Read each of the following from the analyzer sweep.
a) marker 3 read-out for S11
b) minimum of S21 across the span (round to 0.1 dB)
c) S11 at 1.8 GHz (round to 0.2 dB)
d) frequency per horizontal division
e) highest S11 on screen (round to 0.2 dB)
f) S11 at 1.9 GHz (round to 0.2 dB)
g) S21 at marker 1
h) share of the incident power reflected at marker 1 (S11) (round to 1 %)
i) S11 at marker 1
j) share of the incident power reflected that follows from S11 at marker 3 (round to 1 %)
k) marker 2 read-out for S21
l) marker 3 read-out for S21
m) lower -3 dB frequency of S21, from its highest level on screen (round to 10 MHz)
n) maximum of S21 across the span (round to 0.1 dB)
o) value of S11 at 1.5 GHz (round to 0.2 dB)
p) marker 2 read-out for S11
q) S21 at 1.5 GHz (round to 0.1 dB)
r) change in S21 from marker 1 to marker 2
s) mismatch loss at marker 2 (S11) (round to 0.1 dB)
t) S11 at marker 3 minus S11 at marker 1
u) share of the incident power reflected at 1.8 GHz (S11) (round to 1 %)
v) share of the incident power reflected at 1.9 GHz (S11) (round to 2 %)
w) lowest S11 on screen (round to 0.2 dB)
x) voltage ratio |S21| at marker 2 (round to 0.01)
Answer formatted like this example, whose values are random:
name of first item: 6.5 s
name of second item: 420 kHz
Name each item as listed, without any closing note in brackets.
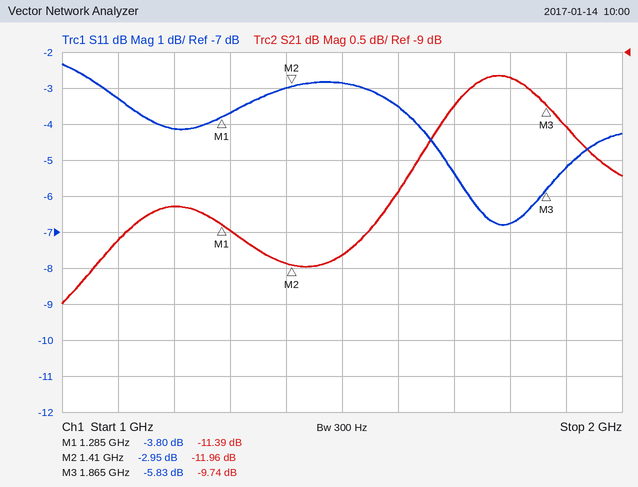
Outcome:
marker 3 read-out for S11: -5.83 dB
minimum of S21 across the span: -12.5 dB
S11 at 1.8 GHz: -6.8 dB
frequency per horizontal division: 100 MHz
highest S11 on screen: -2.4 dB
S11 at 1.9 GHz: -5.2 dB
S21 at marker 1: -11.39 dB
share of the incident power reflected at marker 1 (S11): 42 %
S11 at marker 1: -3.80 dB
share of the incident power reflected that follows from S11 at marker 3: 26 %
marker 2 read-out for S21: -11.96 dB
marker 3 read-out for S21: -9.74 dB
lower -3 dB frequency of S21, from its highest level on screen: 1.02 GHz
maximum of S21 across the span: -9.3 dB
value of S11 at 1.5 GHz: -2.8 dB
marker 2 read-out for S11: -2.95 dB
S21 at 1.5 GHz: -11.8 dB
change in S21 from marker 1 to marker 2: -0.57 dB
mismatch loss at marker 2 (S11): 3.1 dB
S11 at marker 3 minus S11 at marker 1: -2.03 dB
share of the incident power reflected at 1.8 GHz (S11): 21 %
share of the incident power reflected at 1.9 GHz (S11): 30 %
lowest S11 on screen: -6.8 dB
voltage ratio |S21| at marker 2: 0.25
